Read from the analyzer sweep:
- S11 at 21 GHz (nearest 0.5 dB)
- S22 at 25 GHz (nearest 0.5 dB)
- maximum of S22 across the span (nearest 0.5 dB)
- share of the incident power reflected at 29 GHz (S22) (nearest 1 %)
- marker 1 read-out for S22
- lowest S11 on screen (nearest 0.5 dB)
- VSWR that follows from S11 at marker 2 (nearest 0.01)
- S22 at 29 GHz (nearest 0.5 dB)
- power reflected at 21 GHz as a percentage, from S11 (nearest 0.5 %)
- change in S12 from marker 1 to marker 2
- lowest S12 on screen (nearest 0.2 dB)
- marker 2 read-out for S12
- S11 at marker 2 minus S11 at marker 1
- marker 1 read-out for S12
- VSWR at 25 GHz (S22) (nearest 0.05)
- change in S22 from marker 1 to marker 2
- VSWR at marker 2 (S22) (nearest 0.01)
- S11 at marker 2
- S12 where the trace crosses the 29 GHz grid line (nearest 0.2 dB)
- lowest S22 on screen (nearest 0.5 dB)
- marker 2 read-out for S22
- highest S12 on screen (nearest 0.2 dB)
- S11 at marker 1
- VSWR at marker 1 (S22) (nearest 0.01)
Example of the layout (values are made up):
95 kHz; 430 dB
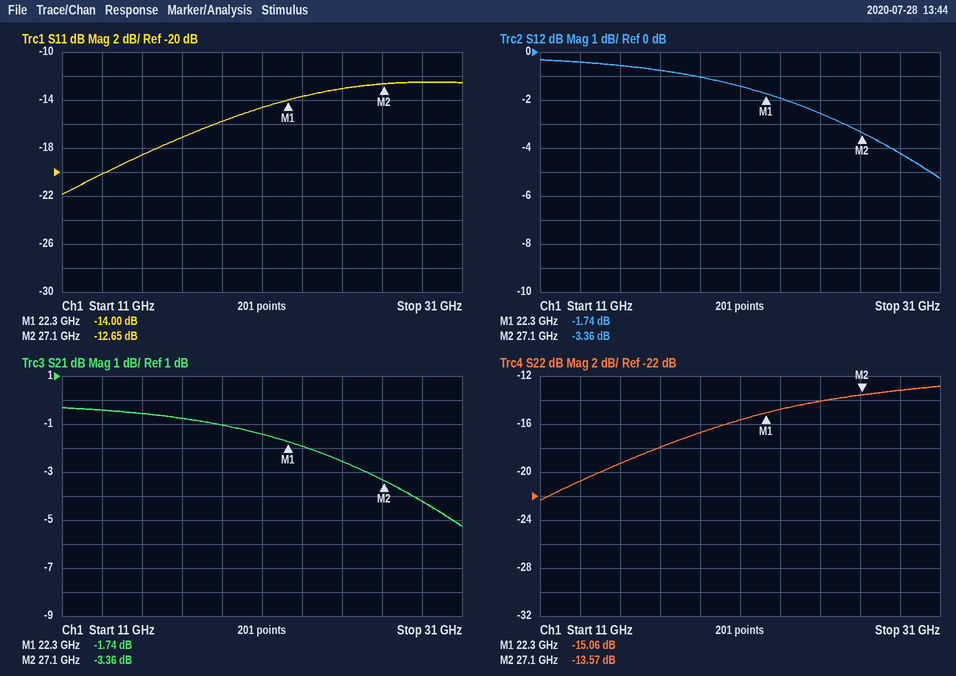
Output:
-14.5 dB; -14.0 dB; -13.0 dB; 5 %; -15.06 dB; -22.0 dB; 1.61; -13.0 dB; 3.5 %; -1.62 dB; -5.2 dB; -3.36 dB; 1.35 dB; -1.74 dB; 1.50; 1.49 dB; 1.53; -12.65 dB; -4.2 dB; -22.5 dB; -13.57 dB; -0.4 dB; -14.00 dB; 1.43
